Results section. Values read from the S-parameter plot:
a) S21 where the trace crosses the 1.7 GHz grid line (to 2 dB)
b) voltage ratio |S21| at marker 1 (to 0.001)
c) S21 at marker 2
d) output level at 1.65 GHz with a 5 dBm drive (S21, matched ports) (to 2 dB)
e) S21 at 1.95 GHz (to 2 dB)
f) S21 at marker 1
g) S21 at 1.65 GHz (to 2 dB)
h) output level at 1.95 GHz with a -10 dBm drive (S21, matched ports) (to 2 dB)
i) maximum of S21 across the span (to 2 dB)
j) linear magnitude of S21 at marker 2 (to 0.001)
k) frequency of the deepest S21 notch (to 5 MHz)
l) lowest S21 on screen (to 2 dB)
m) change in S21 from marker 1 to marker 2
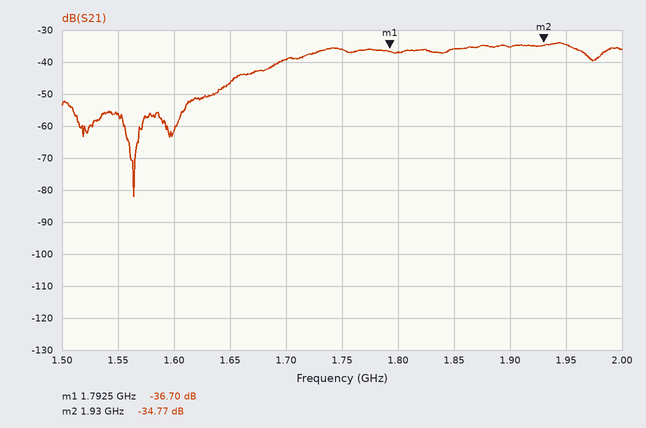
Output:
-40 dB
0.015
-34.77 dB
-42 dBm
-34 dB
-36.70 dB
-46 dB
-44 dBm
-34 dB
0.018
1.565 GHz
-82 dB
1.93 dB
